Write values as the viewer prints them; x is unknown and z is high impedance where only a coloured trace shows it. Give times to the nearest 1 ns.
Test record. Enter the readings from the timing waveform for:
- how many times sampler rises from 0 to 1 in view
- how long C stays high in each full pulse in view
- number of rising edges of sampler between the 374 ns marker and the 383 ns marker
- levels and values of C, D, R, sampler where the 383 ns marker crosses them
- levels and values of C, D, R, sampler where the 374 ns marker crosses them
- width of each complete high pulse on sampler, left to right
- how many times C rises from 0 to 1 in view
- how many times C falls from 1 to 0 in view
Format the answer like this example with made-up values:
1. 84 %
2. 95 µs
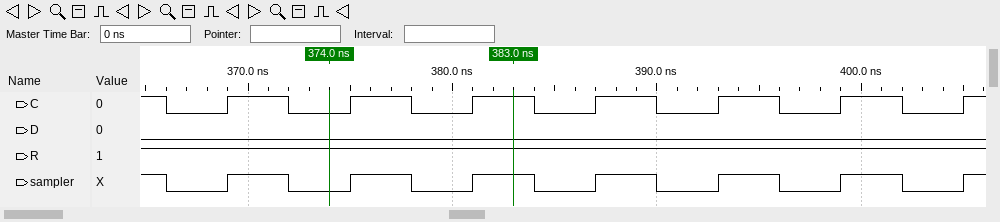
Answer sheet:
1. 7
2. 3 ns, 3 ns, 3 ns, 3 ns, 3 ns, 3 ns
3. 2
4. C=1, D=0, R=1, sampler=1
5. C=0, D=0, R=1, sampler=0
6. 3 ns, 3 ns, 3 ns, 3 ns, 3 ns, 3 ns
7. 7
8. 7
